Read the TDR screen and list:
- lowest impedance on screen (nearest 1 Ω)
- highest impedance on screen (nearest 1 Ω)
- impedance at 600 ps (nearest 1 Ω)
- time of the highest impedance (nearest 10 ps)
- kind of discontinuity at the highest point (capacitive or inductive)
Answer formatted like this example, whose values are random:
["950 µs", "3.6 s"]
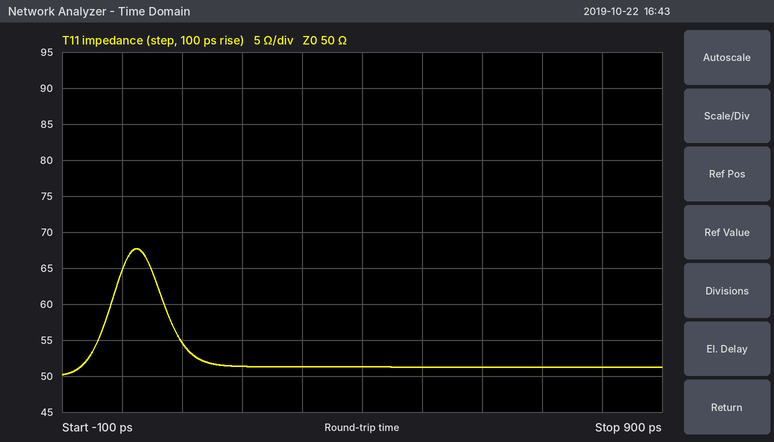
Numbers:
["50 Ω", "68 Ω", "51 Ω", "20 ps", "inductive"]
